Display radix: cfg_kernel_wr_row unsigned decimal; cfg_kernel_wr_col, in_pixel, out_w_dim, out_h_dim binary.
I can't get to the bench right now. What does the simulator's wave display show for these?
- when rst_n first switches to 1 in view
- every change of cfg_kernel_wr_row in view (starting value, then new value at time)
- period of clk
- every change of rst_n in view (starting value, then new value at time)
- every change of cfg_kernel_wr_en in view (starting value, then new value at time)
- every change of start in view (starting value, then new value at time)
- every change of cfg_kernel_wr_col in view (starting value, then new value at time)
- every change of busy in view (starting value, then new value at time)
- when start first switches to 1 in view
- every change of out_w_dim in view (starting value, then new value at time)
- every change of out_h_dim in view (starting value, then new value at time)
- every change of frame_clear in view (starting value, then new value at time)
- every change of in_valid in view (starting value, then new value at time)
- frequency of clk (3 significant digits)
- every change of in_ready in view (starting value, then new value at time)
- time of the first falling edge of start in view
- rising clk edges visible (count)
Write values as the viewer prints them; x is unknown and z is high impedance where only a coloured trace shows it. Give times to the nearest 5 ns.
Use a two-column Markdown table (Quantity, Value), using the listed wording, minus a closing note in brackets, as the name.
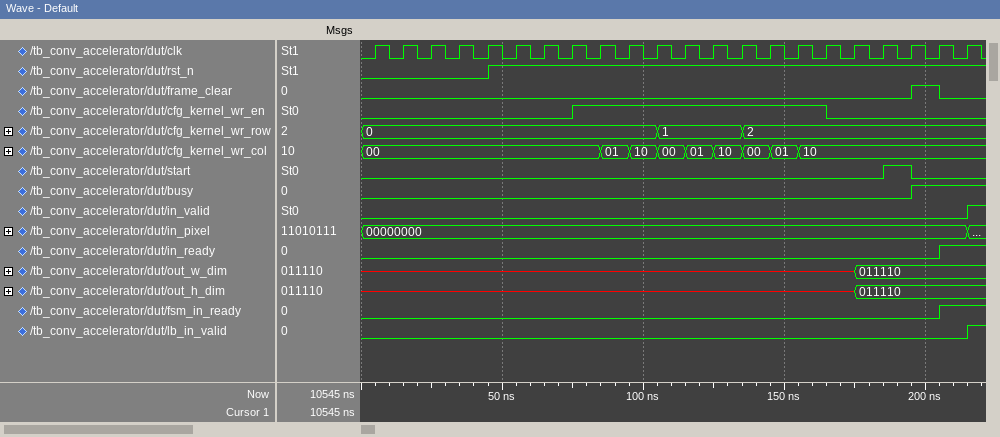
| Quantity | Value |
|---|---|
| when rst_n first switches to 1 in view | 45 ns |
| every change of cfg_kernel_wr_row in view | 0, 1 at 105 ns, 2 at 135 ns |
| period of clk | 10 ns |
| every change of rst_n in view | 0, 1 at 45 ns |
| every change of cfg_kernel_wr_en in view | 0, 1 at 75 ns, 0 at 165 ns |
| every change of start in view | 0, 1 at 185 ns, 0 at 195 ns |
| every change of cfg_kernel_wr_col in view | 00, 01 at 85 ns, 10 at 95 ns, 00 at 105 ns, 01 at 115 ns, 10 at 125 ns, 00 at 135 ns, 01 at 145 ns, 10 at 155 ns |
| every change of busy in view | 0, 1 at 195 ns |
| when start first switches to 1 in view | 185 ns |
| every change of out_w_dim in view | x, 011110 at 175 ns |
| every change of out_h_dim in view | x, 011110 at 175 ns |
| every change of frame_clear in view | 0, 1 at 195 ns, 0 at 205 ns |
| every change of in_valid in view | 0, 1 at 215 ns |
| frequency of clk | 100 MHz |
| every change of in_ready in view | 0, 1 at 205 ns |
| time of the first falling edge of start in view | 195 ns |
| rising clk edges visible | 22 |
